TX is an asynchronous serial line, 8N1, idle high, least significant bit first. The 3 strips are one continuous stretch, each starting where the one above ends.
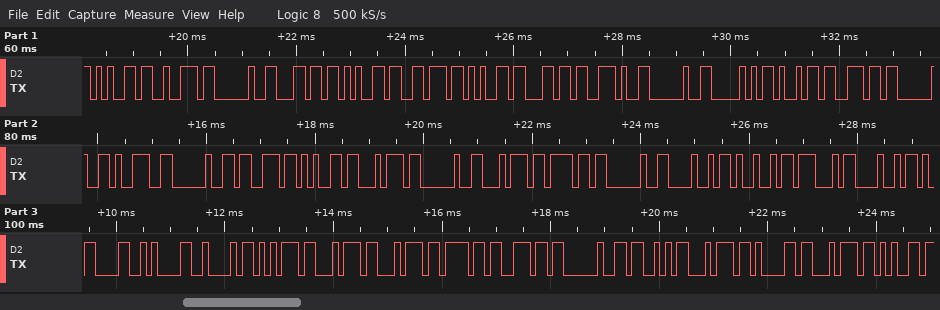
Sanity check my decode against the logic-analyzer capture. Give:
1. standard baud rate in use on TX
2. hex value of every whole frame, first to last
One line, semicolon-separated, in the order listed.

9600 baud; 65 72 20 6C 65 76 65 6C 2E 20 50 69 6E 20 39 20 73 65 74 20 74 6F 20 48 49 47 48 0D 0A 42 75 74 74 6F 6E 20 53 74 61 74 65
